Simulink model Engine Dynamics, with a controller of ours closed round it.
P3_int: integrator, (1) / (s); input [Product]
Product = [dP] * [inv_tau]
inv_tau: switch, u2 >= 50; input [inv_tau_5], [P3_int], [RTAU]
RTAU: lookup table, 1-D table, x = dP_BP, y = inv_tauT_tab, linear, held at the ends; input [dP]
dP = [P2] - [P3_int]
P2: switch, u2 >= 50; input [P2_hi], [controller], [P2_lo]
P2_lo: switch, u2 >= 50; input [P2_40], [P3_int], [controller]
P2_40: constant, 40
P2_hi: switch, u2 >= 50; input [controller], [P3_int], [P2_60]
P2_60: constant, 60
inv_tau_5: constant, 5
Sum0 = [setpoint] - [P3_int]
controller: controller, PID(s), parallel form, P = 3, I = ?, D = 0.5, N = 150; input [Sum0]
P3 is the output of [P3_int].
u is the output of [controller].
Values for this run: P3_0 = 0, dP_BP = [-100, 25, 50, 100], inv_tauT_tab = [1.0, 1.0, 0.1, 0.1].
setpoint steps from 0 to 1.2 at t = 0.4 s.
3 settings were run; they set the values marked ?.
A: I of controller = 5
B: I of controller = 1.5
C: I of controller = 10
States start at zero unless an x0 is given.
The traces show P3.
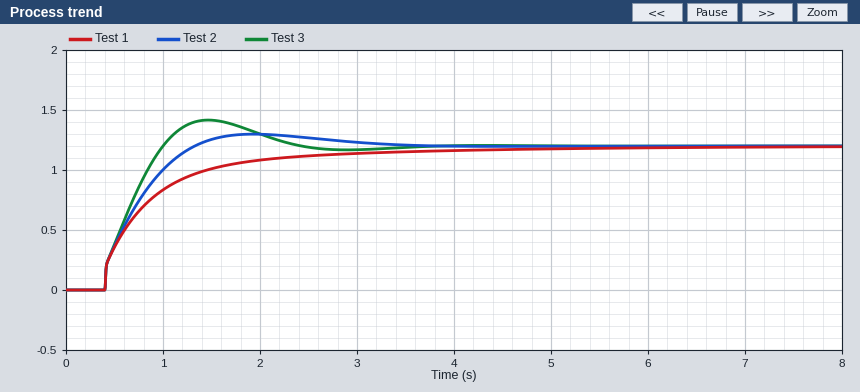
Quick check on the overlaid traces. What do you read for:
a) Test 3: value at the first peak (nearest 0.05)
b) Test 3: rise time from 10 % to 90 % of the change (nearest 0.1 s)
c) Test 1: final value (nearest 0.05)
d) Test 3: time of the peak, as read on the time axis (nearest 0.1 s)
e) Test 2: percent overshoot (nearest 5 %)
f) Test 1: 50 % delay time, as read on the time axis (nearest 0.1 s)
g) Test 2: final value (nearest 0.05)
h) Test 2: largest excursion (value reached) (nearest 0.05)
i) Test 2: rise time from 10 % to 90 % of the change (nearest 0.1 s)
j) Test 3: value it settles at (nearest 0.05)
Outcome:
1.40
0.5 s
1.20
1.5 s
10 %
0.7 s
1.20
1.30
0.7 s
1.20
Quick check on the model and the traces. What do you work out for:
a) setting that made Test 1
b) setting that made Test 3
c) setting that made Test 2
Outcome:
B
C
A
